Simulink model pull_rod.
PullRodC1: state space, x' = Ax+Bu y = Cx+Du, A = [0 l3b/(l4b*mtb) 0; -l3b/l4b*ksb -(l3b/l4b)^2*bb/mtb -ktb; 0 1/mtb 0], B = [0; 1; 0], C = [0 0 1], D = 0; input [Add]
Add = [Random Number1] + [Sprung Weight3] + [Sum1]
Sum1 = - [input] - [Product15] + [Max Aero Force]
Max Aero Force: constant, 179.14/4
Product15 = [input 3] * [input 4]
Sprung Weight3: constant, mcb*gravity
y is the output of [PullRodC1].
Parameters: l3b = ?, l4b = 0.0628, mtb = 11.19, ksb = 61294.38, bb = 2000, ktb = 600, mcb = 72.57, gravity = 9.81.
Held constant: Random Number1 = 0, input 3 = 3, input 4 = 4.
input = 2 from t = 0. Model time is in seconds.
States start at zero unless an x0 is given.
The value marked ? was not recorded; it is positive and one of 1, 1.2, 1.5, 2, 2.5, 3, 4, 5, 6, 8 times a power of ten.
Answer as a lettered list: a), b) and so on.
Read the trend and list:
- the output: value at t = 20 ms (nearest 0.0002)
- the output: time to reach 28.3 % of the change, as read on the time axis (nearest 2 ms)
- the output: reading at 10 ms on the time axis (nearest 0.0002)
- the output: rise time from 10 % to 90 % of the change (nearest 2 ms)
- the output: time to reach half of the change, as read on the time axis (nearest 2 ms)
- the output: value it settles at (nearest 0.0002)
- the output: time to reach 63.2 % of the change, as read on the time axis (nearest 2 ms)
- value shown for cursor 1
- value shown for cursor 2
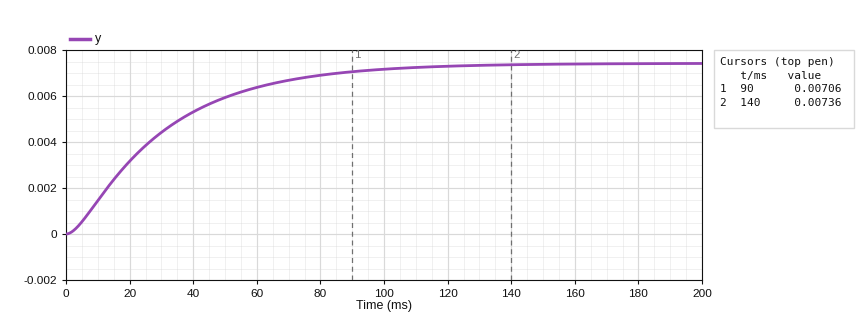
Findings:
a) 0.0032
b) 14 ms
c) 0.0014
d) 64 ms
e) 24 ms
f) 0.0074
g) 32 ms
h) 0.00706
i) 0.00736
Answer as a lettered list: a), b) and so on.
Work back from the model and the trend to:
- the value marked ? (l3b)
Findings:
a) 0.08
